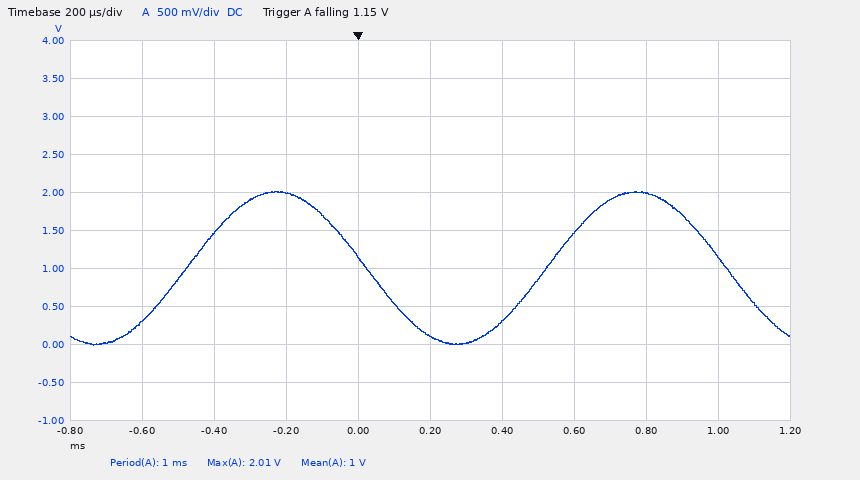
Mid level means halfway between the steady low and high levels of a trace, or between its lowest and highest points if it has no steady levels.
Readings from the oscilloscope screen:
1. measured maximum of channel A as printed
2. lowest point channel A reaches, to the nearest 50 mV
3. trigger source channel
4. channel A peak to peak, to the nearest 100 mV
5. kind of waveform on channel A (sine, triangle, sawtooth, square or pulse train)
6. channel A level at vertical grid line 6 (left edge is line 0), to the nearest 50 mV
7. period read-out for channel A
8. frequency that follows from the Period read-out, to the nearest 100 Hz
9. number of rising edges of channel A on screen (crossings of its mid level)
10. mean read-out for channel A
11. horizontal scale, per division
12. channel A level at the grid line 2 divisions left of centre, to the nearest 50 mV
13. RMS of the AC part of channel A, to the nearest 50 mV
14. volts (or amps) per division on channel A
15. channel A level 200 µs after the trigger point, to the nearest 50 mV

2.01 V
0 mV
channel A
2.00 V
sine
300 mV
1 ms
1.0 kHz
2
1 V
200 µs
2.00 V
700 mV
500 mV
100 mV
